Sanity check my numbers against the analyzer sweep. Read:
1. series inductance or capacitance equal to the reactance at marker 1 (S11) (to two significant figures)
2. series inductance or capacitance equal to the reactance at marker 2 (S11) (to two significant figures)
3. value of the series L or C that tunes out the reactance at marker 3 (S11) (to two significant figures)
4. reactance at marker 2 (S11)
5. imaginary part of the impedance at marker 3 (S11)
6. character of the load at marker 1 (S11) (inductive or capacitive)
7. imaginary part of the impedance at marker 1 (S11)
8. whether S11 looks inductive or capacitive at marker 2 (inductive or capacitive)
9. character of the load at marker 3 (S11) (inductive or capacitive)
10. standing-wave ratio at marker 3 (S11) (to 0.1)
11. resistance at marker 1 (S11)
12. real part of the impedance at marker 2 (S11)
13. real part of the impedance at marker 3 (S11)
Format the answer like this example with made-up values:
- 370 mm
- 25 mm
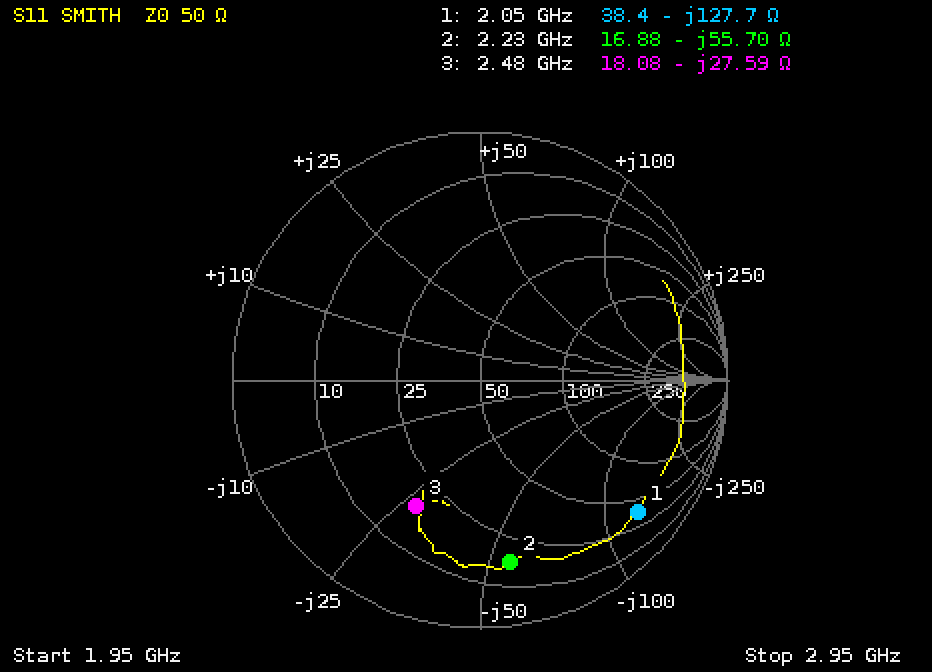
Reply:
- 610 fF
- 1.3 pF
- 1.8 nH
- -55.70 Ω
- -27.59 Ω
- capacitive
- -127.7 Ω
- capacitive
- capacitive
- 3.7
- 38.4 Ω
- 16.88 Ω
- 18.08 Ω
